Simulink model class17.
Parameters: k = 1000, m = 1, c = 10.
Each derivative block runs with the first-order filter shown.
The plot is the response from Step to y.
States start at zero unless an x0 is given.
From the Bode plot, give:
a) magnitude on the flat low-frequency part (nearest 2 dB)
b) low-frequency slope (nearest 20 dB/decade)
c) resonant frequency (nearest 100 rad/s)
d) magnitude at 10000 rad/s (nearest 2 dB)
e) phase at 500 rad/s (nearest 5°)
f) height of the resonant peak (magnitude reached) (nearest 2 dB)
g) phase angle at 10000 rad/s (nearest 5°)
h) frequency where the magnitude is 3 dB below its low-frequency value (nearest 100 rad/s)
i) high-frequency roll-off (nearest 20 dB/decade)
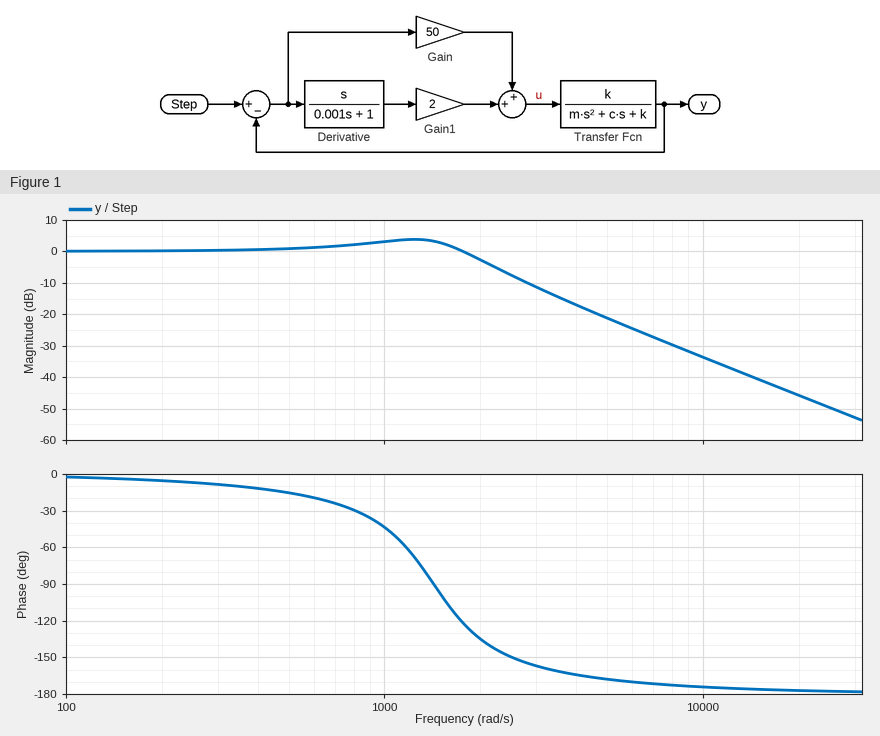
0 dB
0 dB/decade
1200 rad/s
-34 dB
-15°
4 dB
-175°
2000 rad/s
-40 dB/decade
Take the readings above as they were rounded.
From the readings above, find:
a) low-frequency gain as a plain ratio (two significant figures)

1.0
